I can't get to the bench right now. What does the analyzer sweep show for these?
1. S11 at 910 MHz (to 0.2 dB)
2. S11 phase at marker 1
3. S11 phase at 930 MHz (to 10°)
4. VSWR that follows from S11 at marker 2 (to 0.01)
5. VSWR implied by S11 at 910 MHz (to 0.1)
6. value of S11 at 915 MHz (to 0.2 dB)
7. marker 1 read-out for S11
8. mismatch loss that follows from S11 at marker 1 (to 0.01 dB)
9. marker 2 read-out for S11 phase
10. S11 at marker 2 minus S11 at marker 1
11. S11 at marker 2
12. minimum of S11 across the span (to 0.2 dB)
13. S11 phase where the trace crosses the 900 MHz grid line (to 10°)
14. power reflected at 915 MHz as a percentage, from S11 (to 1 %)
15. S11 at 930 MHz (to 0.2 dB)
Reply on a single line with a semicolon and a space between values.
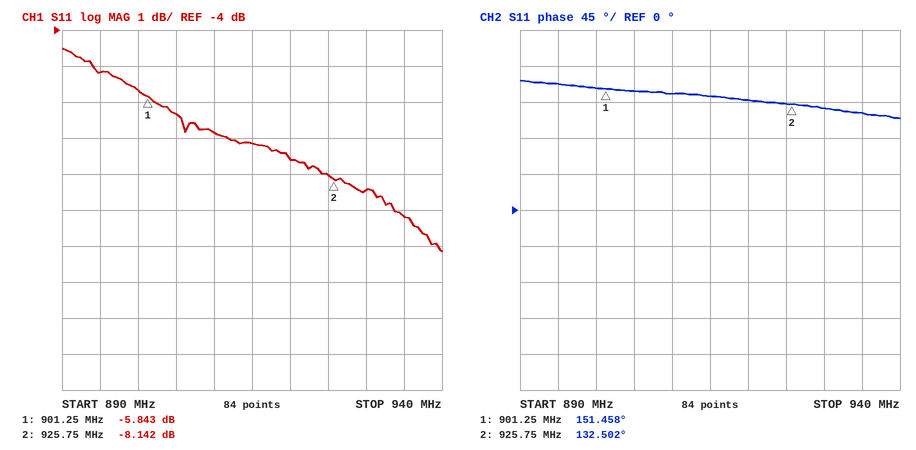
-6.8 dB; 151.458°; 130°; 2.29; 2.7; -7.2 dB; -5.843 dB; 1.31 dB; 132.502°; -2.299 dB; -8.142 dB; -10.2 dB; 150°; 19 %; -8.4 dB
